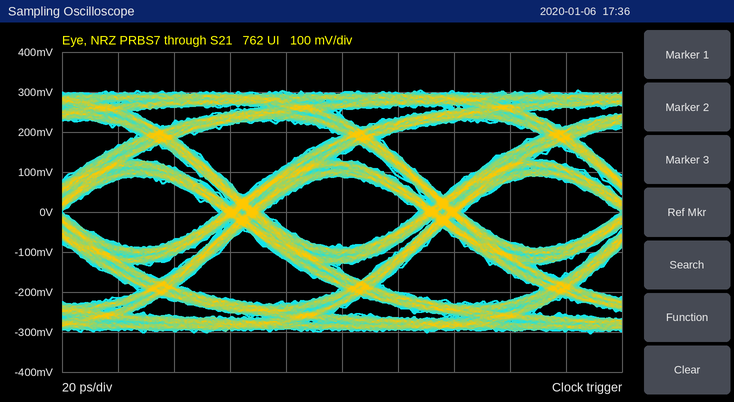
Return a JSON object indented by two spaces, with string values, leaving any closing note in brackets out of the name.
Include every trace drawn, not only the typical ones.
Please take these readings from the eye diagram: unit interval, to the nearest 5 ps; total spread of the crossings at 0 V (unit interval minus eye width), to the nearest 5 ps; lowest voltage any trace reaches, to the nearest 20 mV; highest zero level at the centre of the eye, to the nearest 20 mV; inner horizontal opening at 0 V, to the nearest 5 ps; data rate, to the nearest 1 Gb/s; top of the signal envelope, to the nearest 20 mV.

{
  "unit interval, to the nearest 5 ps": "70 ps",
  "total spread of the crossings at 0 V (unit interval minus eye width), to the nearest 5 ps": "15 ps",
  "lowest voltage any trace reaches, to the nearest 20 mV": "-300 mV",
  "highest zero level at the centre of the eye, to the nearest 20 mV": "-80 mV",
  "inner horizontal opening at 0 V, to the nearest 5 ps": "55 ps",
  "data rate, to the nearest 1 Gb/s": "14 Gb/s",
  "top of the signal envelope, to the nearest 20 mV": "300 mV"
}
